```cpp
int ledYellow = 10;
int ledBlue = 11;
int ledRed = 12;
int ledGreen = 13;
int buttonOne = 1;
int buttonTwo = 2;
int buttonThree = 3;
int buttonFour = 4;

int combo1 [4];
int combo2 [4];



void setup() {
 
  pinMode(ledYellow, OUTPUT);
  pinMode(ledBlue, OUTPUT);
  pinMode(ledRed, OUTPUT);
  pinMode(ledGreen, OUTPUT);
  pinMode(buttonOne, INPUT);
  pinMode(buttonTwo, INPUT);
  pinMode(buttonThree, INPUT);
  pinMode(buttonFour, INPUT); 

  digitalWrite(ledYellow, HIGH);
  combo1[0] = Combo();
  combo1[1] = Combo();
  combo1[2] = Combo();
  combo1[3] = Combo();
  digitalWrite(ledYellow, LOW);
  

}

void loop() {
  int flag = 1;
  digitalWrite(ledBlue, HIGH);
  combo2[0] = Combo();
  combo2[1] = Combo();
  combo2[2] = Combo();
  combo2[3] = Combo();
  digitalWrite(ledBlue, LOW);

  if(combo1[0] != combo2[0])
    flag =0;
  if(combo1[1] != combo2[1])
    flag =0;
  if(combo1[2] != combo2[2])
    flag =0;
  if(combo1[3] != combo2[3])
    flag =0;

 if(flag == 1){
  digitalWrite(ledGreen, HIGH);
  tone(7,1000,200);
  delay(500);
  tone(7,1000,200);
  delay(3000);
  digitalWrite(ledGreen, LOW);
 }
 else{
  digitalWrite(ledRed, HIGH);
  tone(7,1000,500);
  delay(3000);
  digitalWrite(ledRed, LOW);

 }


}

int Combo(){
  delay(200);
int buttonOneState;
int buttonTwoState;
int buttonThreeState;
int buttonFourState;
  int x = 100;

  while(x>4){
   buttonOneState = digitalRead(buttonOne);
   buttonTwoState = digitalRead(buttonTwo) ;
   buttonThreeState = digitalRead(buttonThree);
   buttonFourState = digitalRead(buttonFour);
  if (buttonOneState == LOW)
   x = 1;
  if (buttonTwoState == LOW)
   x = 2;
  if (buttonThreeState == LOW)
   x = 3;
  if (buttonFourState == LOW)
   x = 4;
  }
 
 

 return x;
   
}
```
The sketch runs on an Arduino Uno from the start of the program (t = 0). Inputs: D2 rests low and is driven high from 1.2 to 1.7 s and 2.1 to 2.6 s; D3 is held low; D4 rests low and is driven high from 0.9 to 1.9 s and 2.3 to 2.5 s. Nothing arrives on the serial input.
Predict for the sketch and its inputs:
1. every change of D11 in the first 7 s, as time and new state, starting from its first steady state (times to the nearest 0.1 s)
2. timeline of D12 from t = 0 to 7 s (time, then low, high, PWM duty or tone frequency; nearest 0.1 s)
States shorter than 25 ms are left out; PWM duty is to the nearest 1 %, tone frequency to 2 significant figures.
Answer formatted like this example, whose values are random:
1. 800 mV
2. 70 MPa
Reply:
1. 0 s low; 0.8 s high; 1.6 s low; 4.6 s high; 5.4 s low
2. 0 s low; 1.6 s high; 4.6 s low
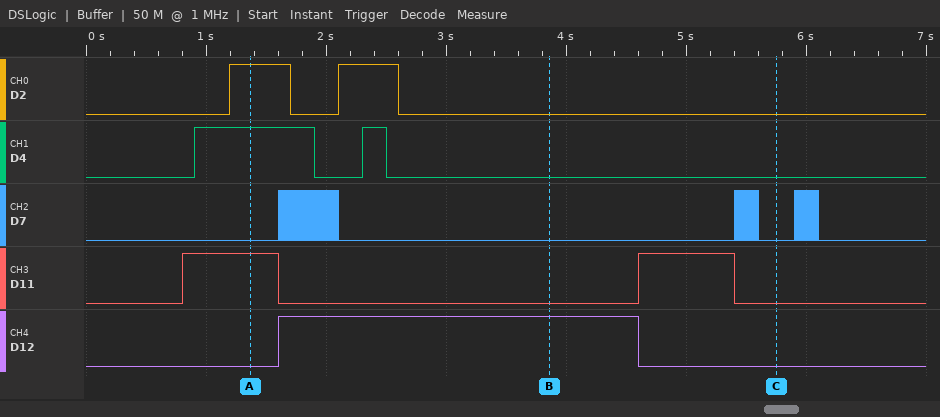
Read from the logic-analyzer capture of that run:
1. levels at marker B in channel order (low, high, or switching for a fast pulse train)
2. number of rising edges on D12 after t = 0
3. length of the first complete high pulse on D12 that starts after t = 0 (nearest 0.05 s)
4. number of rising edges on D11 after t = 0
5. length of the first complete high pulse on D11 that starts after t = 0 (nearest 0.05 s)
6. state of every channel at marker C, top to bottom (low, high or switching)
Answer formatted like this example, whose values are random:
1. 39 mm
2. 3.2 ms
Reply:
1. D2 low, D4 low, D7 low, D11 low, D12 high
2. 1
3. 3.00 s
4. 2
5. 0.80 s
6. D2 low, D4 low, D7 low, D11 low, D12 low
